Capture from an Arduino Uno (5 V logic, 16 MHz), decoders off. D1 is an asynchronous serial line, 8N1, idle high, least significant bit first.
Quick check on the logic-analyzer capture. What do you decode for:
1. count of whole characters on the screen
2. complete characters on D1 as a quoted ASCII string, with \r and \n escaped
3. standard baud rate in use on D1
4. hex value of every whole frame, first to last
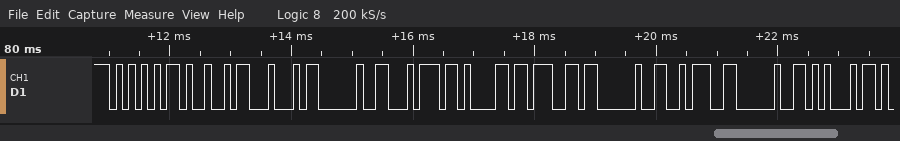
11
"UID tag : E"
9600 baud
55 49 44 20 74 61 67 20 3A 20 45
